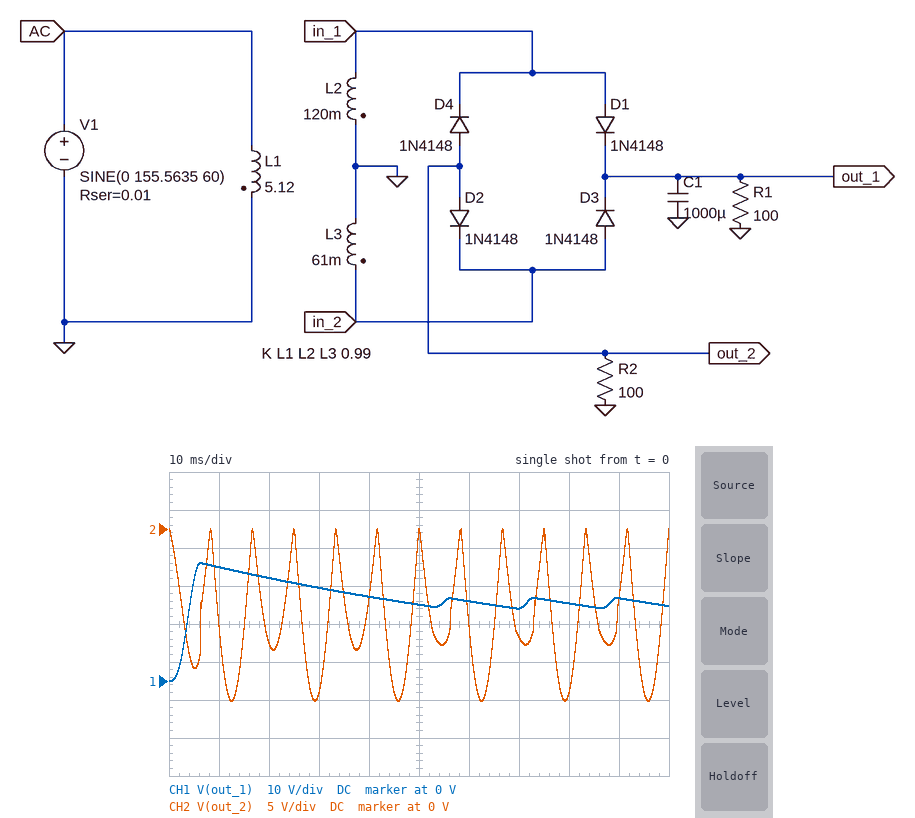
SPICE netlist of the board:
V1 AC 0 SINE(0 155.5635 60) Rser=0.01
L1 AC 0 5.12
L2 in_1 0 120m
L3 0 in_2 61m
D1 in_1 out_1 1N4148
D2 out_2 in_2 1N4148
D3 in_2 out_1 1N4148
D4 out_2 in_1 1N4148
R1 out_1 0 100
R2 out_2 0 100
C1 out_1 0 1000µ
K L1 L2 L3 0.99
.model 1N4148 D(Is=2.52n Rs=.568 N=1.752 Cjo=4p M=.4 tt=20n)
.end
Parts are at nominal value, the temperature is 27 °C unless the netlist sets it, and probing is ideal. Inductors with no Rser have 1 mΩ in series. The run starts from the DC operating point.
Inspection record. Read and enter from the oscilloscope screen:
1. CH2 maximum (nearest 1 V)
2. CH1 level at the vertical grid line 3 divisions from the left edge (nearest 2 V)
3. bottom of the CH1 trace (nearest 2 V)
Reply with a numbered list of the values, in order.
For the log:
1. 0 V
2. 24 V
3. 0 V
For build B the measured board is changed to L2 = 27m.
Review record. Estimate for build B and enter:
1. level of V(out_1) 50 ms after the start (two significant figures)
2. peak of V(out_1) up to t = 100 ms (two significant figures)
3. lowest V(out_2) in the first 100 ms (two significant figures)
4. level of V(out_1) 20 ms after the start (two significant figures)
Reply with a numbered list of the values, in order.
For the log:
1. 15 V
2. 17 V
3. -17 V
4. 16 V
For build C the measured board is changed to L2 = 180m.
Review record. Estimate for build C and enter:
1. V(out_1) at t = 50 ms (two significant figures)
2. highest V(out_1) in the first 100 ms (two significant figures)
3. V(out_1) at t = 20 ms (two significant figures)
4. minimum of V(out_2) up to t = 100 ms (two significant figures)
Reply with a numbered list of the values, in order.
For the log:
1. 25 V
2. 39 V
3. 34 V
4. -28 V
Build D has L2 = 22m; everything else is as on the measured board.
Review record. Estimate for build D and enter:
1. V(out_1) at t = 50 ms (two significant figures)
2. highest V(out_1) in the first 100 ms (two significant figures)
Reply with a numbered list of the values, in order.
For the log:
1. 15 V
2. 18 V
